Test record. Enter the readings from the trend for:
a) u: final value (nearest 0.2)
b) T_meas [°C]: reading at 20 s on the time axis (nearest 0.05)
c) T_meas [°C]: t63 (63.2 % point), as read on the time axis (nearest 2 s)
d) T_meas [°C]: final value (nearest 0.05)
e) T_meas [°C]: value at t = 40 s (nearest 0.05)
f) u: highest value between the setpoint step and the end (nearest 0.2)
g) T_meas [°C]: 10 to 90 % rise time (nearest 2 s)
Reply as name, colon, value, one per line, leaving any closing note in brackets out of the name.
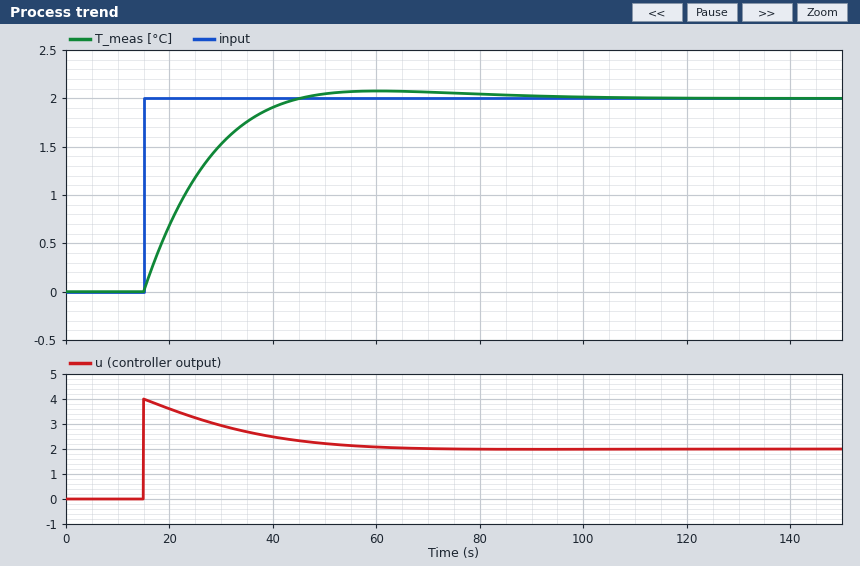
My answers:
u: final value: 2.0
T_meas [°C]: reading at 20 s on the time axis: 0.70
T_meas [°C]: t63 (63.2 % point), as read on the time axis: 26 s
T_meas [°C]: final value: 2.00
T_meas [°C]: value at t = 40 s: 1.90
u: highest value between the setpoint step and the end: 4.0
T_meas [°C]: 10 to 90 % rise time: 20 s
